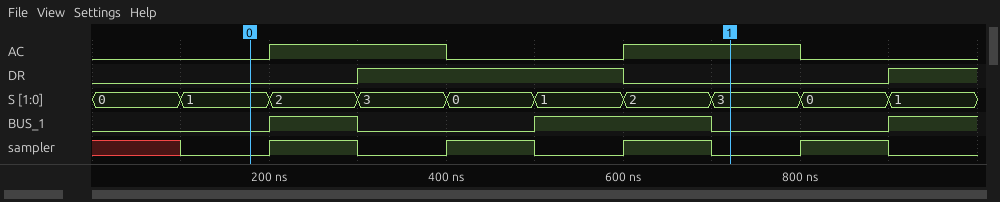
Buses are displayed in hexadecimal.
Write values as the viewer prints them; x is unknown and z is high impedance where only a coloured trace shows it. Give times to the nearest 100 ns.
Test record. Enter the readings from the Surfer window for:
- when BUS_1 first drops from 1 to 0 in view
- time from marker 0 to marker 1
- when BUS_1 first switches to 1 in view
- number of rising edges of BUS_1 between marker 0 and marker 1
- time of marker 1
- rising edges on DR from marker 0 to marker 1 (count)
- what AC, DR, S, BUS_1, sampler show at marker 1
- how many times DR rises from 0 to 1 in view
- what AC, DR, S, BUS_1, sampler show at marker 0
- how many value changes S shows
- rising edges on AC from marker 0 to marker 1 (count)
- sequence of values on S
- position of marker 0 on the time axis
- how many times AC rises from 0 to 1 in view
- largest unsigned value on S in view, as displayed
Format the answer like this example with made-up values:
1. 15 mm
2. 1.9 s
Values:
1. 300 ns
2. 500 ns
3. 200 ns
4. 2
5. 700 ns
6. 1
7. AC=1, DR=0, S=3, BUS_1=0, sampler=0
8. 2
9. AC=0, DR=0, S=1, BUS_1=0, sampler=0
10. 9
11. 2
12. 0, 1, 2, 3, 0, 1, 2, 3, 0, 1
13. 200 ns
14. 2
15. 3
